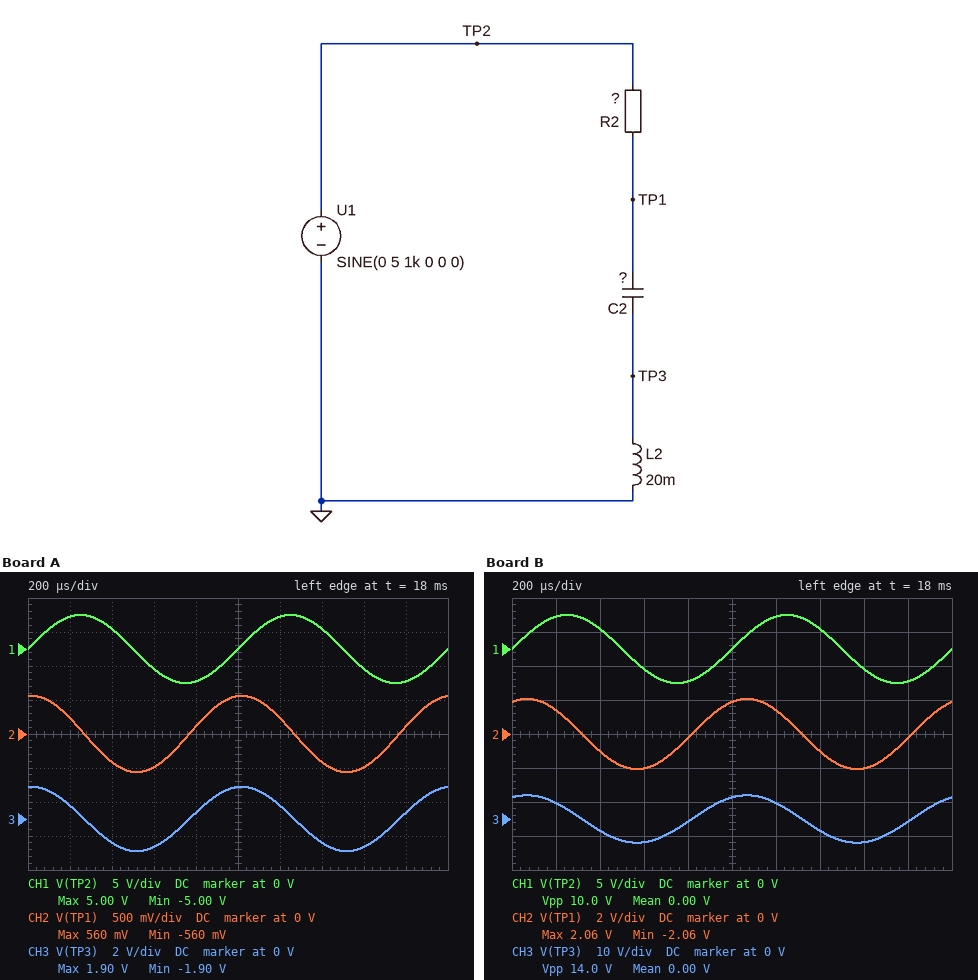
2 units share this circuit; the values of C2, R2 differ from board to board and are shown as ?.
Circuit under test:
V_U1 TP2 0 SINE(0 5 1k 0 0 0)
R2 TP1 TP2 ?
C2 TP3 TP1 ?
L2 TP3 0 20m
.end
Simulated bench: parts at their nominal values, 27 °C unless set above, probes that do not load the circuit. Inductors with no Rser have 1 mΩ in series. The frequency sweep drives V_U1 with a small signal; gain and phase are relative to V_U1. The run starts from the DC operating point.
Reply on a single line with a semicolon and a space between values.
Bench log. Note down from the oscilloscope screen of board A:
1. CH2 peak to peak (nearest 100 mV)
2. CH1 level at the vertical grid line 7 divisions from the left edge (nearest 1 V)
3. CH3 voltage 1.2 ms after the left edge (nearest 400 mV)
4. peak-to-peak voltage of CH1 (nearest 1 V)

1.1 V; 3 V; 800 mV; 10 V
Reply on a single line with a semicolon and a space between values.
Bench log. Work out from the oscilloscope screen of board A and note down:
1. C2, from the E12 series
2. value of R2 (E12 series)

1.8 µF; 330 Ω
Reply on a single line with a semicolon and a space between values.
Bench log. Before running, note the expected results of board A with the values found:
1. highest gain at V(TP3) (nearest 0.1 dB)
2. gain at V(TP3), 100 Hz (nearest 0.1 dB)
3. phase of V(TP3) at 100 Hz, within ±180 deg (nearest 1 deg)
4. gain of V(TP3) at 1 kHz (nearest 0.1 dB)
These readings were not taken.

0 dB; -37.4 dB; 159 deg; -8.4 dB
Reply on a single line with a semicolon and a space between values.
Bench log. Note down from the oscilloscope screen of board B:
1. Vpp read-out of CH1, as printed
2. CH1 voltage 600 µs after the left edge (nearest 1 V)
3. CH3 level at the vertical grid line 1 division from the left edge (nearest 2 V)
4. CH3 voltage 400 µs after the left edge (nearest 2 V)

10.0 V; -3 V; 4 V; -4 V
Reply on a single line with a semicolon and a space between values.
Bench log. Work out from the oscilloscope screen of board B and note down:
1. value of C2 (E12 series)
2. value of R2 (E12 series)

1.8 µF; 82 Ω
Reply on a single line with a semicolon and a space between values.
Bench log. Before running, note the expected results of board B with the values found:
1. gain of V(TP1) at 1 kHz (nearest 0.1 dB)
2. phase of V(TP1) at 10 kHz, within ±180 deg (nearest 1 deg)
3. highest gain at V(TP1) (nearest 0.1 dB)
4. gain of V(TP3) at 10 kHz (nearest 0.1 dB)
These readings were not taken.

-7.7 dB; 4 deg; 0 dB; 0 dB
